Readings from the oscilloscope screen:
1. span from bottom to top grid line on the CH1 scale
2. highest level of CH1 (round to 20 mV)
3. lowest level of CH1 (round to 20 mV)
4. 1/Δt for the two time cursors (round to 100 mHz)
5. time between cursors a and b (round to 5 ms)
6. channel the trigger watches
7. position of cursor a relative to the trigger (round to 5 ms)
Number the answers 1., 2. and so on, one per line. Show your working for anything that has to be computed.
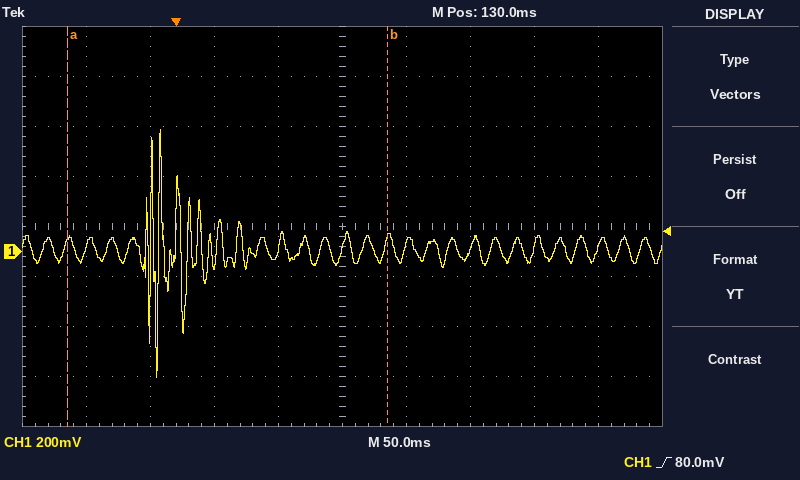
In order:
1. 1.6 V
2. 480 mV
3. -500 mV
4. 1 / 250 ms ≈ 4.0 Hz
5. 250 ms
6. CH1
7. -85 ms
